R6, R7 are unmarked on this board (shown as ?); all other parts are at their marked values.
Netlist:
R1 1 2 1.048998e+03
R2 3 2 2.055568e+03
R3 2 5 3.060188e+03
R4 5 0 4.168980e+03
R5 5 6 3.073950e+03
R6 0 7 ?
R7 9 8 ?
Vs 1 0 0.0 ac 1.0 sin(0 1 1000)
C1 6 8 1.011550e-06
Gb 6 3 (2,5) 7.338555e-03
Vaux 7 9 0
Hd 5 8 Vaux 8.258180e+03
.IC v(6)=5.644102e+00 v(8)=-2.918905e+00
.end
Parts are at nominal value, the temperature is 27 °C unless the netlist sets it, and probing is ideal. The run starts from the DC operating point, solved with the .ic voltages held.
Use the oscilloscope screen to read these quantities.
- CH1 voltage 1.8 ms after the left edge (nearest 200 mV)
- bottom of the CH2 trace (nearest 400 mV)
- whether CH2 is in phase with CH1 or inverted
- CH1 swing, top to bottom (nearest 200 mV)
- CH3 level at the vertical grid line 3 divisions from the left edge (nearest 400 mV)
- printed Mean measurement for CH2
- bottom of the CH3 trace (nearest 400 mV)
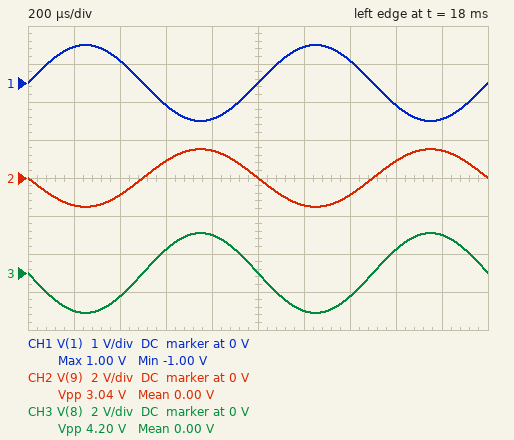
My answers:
-1.0 V
-1.6 V
inverted
2.0 V
1.2 V
0.00 V
-2.0 V
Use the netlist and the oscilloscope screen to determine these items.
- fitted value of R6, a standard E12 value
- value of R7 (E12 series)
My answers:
3.9 kΩ
1.5 kΩ
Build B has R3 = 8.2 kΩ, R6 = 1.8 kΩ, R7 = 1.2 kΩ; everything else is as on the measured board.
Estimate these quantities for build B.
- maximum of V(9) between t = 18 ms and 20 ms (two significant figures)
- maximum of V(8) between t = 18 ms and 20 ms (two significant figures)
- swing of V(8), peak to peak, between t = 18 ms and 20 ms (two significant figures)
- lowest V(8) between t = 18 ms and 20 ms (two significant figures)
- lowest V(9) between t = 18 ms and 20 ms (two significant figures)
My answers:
330 mV
550 mV
1.1 V
-550 mV
-330 mV
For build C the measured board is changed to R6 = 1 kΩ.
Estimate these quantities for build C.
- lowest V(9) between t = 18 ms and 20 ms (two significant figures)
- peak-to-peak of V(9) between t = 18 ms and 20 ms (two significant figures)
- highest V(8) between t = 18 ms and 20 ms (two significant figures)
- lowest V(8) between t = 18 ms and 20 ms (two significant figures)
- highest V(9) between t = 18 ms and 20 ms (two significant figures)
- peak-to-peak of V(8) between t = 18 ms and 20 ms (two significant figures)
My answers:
-160 mV
330 mV
410 mV
-410 mV
160 mV
820 mV
